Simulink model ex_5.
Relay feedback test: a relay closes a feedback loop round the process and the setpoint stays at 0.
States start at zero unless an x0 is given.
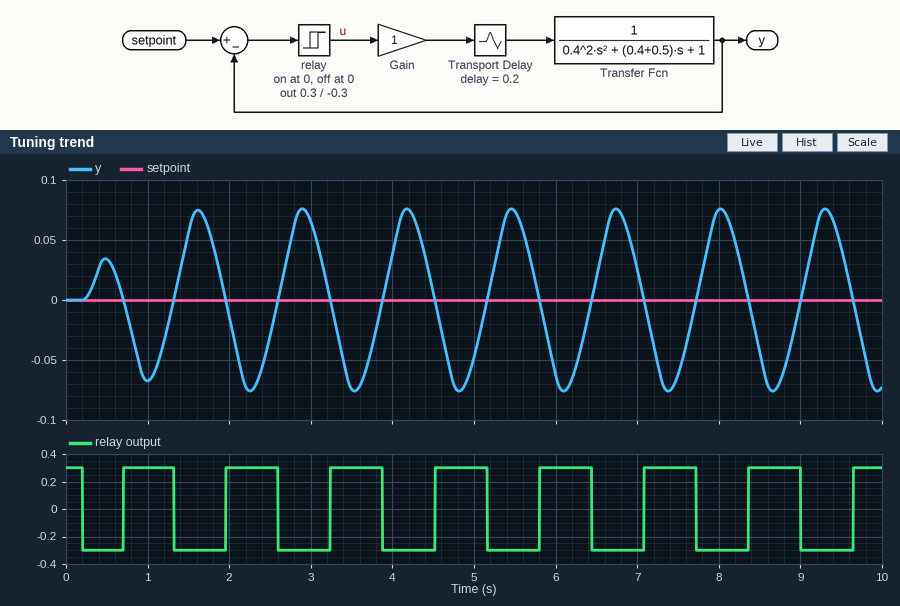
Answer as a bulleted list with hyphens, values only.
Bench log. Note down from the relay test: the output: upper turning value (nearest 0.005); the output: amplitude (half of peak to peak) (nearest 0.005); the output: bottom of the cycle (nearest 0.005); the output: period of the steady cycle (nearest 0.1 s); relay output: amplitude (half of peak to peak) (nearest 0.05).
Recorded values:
- 0.075
- 0.075
- -0.075
- 1.3 s
- 0.30
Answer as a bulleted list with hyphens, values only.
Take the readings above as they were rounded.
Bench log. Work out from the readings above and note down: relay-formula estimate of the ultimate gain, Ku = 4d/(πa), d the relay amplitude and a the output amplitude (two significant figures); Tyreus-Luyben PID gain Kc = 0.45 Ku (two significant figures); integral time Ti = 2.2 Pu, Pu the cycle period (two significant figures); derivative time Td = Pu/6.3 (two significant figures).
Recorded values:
- 5.1
- 2.3
- 2.9 s
- 0.21 s
